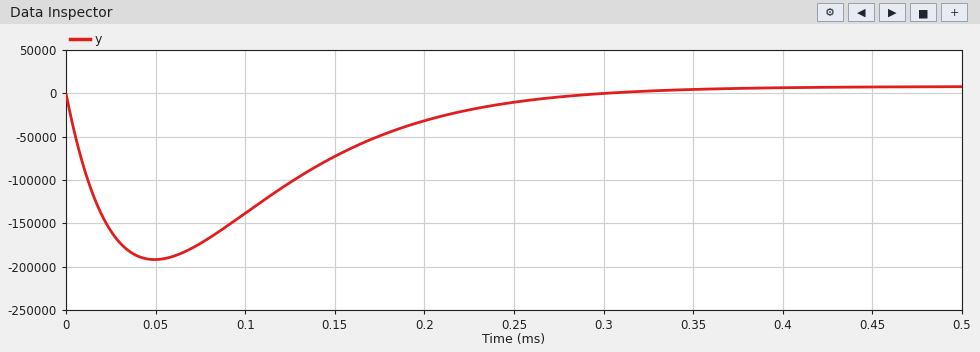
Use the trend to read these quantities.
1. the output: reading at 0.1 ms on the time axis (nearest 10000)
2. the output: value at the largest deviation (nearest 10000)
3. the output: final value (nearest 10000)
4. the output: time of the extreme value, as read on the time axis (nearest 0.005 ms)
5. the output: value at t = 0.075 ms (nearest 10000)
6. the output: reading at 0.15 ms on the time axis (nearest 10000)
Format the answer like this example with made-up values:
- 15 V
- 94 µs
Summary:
- -140000
- -190000
- 10000
- 0.050 ms
- -170000
- -70000
